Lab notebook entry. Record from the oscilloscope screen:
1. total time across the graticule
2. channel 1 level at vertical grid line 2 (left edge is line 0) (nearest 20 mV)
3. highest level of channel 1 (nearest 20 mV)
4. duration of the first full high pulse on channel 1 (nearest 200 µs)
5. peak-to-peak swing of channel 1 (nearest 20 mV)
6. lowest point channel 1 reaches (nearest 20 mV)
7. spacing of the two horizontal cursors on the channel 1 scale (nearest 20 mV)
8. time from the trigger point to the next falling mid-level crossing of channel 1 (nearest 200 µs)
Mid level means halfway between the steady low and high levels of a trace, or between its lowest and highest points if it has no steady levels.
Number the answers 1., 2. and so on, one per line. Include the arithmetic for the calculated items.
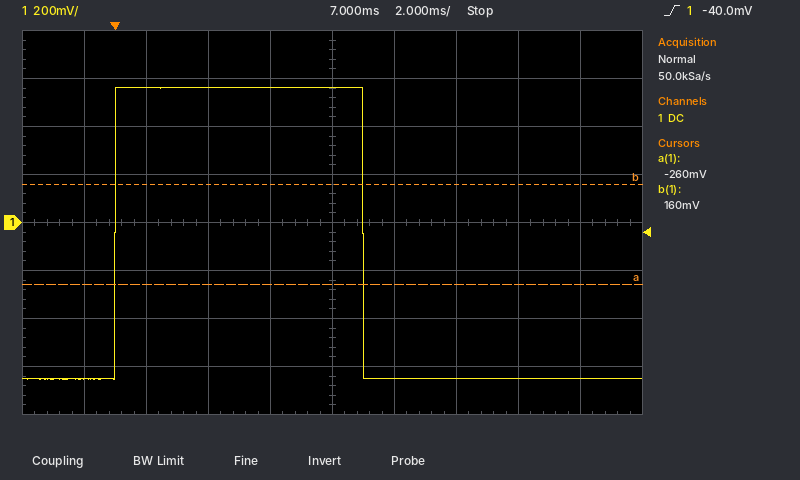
1. 20 ms
2. 560 mV
3. 560 mV
4. 8.0 ms
5. 560 mV − (-660 mV) = 1.22 V
6. -660 mV
7. 420 mV
8. 8.0 ms
